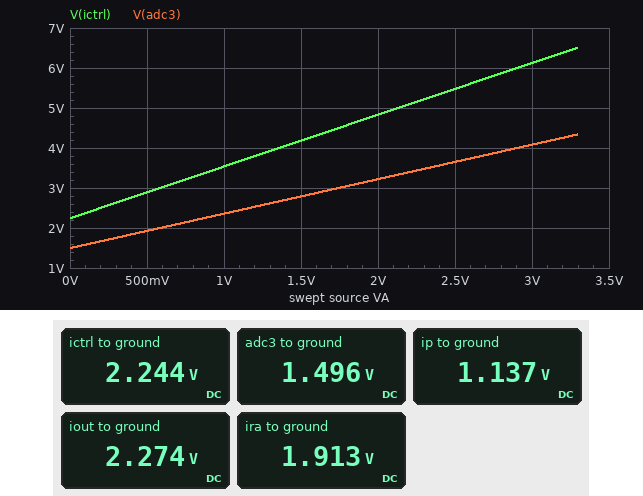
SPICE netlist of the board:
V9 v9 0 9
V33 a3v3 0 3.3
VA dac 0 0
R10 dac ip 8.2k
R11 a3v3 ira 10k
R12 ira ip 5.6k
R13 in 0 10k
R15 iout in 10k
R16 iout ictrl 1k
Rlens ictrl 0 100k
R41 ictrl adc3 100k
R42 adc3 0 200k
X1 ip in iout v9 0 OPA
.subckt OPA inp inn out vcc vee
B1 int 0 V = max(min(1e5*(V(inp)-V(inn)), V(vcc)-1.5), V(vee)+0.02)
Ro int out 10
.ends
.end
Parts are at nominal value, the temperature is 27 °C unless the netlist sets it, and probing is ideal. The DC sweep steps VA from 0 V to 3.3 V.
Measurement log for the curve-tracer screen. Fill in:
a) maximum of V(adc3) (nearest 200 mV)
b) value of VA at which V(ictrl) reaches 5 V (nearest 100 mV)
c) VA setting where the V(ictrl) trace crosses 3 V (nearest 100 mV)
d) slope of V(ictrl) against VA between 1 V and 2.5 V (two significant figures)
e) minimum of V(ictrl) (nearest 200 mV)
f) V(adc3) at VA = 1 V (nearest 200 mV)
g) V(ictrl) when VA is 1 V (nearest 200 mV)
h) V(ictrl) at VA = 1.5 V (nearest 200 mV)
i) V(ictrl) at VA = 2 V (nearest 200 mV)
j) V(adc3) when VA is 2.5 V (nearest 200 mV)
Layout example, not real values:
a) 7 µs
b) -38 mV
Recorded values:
a) 4.4 V
b) 2.1 V
c) 600 mV
d) 1.3 V/V
e) 2.2 V
f) 2.4 V
g) 3.6 V
h) 4.2 V
i) 4.8 V
j) 3.6 V
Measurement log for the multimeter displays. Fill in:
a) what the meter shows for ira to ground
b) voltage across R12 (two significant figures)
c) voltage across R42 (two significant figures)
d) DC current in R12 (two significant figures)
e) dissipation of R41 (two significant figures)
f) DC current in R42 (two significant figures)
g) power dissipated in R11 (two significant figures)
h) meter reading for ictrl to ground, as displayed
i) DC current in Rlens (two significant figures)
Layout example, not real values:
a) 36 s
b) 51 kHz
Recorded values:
a) 1.913 V
b) 780 mV
c) 1.5 V
d) 140 µA
e) 5.6 µW
f) 7.5 µA
g) 190 µW
h) 2.244 V
i) 22 µA
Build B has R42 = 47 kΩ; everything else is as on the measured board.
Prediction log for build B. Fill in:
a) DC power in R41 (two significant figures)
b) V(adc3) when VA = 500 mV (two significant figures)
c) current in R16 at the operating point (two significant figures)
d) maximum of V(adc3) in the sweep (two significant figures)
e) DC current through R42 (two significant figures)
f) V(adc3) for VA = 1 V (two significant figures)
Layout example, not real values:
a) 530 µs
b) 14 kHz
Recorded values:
a) 23 µW
b) 920 mV
c) 38 µA
d) 2.1 V
e) 15 µA
f) 1.1 V
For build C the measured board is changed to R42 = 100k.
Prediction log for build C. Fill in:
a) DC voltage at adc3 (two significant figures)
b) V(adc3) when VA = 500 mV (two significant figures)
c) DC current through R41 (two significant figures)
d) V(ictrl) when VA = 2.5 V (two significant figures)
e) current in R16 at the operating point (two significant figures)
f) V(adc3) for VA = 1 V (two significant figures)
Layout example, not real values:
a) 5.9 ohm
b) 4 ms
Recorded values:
a) 1.1 V
b) 1.4 V
c) 11 µA
d) 5.5 V
e) 34 µA
f) 1.8 V
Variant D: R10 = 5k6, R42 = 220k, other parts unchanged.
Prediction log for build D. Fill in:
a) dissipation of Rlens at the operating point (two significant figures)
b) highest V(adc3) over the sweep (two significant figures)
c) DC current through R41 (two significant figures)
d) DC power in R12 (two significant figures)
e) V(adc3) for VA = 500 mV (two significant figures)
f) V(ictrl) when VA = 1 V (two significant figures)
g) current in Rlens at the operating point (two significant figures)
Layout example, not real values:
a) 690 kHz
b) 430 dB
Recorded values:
a) 30 µW
b) 4.5 V
c) 5.4 µA
d) 140 µW
e) 1.7 V
f) 3.2 V
g) 17 µA
